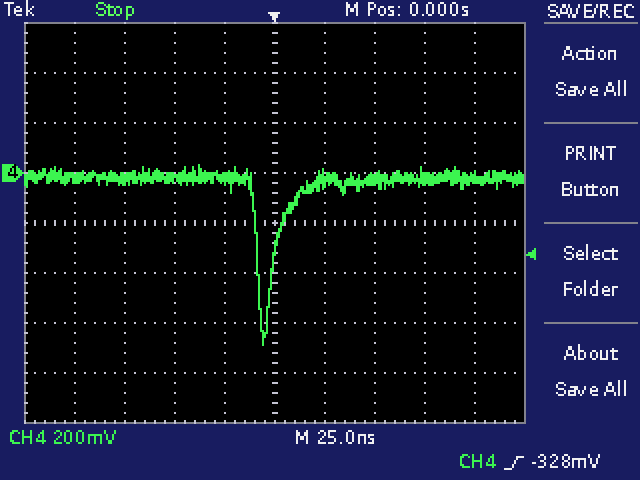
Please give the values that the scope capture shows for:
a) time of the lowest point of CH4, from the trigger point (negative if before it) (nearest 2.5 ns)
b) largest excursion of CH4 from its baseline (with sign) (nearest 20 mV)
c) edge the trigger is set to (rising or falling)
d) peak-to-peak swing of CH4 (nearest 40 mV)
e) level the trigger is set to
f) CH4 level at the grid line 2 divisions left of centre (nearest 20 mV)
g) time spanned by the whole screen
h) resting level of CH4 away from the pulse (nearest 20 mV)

-5.0 ns
-660 mV
rising
720 mV
-328 mV
-20 mV
250 ns
-20 mV
